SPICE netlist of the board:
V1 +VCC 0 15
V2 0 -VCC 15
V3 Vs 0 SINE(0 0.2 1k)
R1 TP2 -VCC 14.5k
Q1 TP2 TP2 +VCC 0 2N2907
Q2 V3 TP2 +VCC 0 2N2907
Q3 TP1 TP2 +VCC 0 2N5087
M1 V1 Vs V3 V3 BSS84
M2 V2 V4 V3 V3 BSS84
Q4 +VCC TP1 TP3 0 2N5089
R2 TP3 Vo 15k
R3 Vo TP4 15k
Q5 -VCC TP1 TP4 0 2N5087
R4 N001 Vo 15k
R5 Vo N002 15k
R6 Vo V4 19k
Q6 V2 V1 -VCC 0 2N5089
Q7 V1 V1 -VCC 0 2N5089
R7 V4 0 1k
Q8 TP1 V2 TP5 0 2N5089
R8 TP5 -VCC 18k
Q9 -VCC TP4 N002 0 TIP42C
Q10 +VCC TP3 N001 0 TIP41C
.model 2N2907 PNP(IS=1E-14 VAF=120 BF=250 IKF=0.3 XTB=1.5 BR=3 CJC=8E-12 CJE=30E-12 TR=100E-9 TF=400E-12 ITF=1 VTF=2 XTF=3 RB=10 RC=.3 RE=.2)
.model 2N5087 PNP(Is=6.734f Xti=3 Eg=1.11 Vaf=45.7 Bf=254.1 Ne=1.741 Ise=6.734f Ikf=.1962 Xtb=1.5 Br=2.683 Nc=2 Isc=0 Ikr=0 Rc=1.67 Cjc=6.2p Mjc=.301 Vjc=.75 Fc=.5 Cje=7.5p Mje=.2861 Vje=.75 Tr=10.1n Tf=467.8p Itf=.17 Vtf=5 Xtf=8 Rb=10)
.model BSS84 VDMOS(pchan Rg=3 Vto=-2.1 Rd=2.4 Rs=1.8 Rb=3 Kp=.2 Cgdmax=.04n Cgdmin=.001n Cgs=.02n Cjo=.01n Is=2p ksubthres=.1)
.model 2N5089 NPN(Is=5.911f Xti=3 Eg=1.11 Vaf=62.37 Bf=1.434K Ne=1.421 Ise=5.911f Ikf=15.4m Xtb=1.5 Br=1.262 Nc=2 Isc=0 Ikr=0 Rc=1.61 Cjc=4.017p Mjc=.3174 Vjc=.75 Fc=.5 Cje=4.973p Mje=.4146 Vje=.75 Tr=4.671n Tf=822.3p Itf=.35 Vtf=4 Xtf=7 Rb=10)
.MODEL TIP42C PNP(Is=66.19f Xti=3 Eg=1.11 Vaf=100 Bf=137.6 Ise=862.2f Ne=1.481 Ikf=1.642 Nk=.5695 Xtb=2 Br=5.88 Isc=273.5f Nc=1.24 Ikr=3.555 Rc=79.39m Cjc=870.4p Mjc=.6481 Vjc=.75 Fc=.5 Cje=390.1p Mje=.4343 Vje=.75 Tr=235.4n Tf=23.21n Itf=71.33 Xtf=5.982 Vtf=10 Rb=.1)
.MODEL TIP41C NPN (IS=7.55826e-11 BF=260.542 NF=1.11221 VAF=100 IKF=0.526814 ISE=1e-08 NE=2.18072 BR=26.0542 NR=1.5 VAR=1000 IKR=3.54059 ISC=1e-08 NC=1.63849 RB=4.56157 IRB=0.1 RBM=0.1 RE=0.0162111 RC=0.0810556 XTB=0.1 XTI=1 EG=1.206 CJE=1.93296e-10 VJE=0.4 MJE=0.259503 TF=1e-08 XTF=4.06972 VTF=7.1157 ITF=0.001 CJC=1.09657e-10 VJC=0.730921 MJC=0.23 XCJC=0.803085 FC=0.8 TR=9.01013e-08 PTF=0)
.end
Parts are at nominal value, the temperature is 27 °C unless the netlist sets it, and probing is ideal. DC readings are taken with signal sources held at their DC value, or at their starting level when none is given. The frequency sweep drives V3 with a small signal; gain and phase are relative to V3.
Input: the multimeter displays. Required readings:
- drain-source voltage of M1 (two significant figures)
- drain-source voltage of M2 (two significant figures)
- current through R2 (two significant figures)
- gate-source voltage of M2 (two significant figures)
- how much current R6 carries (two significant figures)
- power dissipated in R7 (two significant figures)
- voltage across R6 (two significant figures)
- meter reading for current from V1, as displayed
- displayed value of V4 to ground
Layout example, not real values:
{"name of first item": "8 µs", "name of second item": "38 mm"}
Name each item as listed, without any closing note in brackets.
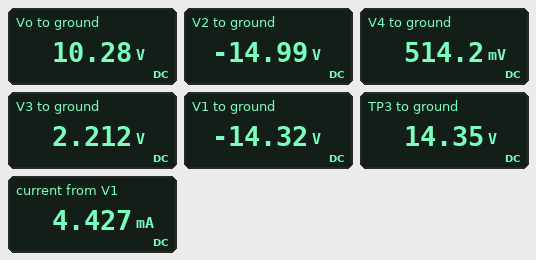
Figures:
{"drain-source voltage of M1": "-17 V", "drain-source voltage of M2": "-17 V", "current through R2": "270 µA", "gate-source voltage of M2": "-1.7 V", "how much current R6 carries": "510 µA", "power dissipated in R7": "260 µW", "voltage across R6": "9.8 V", "meter reading for current from V1, as displayed": "4.427 mA", "displayed value of V4 to ground": "514.2 mV"}
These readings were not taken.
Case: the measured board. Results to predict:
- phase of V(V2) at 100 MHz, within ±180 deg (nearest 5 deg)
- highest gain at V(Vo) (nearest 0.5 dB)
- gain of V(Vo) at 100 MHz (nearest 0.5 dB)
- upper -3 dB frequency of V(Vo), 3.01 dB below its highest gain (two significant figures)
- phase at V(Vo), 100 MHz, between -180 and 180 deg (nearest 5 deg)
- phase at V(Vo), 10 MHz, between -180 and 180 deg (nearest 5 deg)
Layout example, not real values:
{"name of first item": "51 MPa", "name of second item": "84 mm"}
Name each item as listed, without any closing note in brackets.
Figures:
{"phase of V(V2) at 100 MHz, within ±180 deg": "100 deg", "highest gain at V(Vo)": "-17.5 dB", "gain of V(Vo) at 100 MHz": "-18.5 dB", "upper -3 dB frequency of V(Vo), 3.01 dB below its highest gain": "2.1 GHz", "phase at V(Vo), 100 MHz, between -180 and 180 deg": "-5 deg", "phase at V(Vo), 10 MHz, between -180 and 180 deg": "35 deg"}
